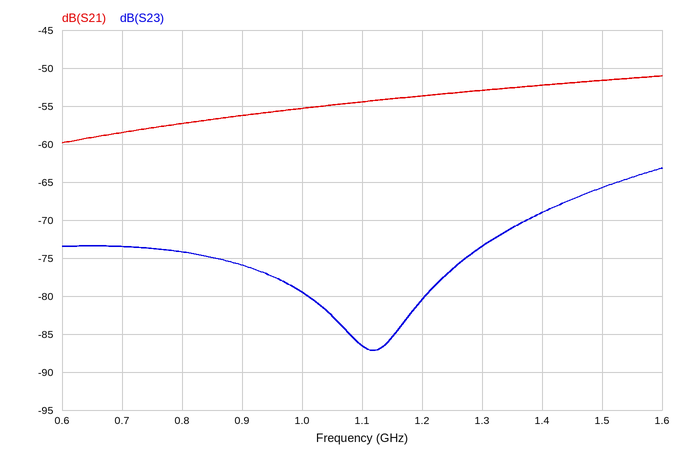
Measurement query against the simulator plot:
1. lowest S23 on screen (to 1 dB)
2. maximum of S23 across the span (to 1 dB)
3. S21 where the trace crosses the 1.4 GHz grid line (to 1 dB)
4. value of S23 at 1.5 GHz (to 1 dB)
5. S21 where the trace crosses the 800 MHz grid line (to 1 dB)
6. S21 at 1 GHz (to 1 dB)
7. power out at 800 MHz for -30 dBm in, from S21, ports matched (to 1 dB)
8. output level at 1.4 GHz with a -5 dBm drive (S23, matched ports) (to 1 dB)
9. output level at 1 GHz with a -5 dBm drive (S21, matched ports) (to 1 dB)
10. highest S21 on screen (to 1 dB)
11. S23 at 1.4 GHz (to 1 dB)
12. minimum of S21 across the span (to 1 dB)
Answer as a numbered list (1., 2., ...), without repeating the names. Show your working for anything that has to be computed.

1. -87 dB
2. -63 dB
3. -52 dB
4. -66 dB
5. -57 dB
6. -55 dB
7. -30 dBm + (-57 dB) = -87 dBm
8. -5 dBm + (-69 dB) = -74 dBm
9. -5 dBm + (-55 dB) = -60 dBm
10. -51 dB
11. -69 dB
12. -60 dB
